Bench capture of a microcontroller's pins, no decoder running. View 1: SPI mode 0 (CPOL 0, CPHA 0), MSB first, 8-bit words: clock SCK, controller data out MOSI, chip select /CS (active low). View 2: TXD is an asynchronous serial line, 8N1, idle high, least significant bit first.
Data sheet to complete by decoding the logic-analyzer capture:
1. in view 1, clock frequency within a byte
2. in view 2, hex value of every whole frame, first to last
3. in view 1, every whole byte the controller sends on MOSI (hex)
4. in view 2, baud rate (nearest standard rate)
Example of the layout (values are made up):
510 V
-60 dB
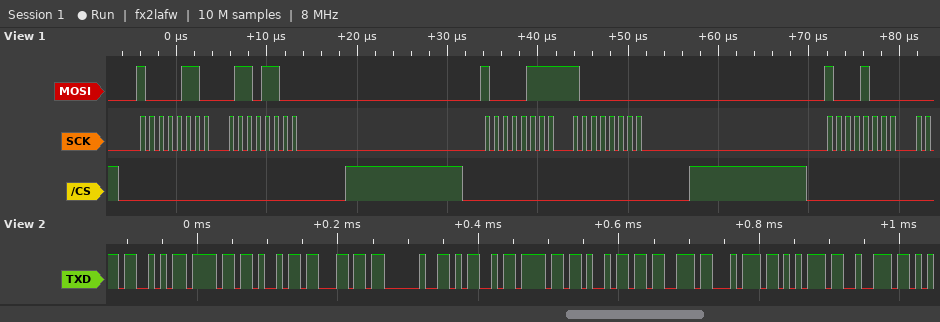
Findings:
1 MHz
53 6F 69 6C 20 4D 6F 69 73 74 75 72
86 6C 87 80 88
115200 baud
